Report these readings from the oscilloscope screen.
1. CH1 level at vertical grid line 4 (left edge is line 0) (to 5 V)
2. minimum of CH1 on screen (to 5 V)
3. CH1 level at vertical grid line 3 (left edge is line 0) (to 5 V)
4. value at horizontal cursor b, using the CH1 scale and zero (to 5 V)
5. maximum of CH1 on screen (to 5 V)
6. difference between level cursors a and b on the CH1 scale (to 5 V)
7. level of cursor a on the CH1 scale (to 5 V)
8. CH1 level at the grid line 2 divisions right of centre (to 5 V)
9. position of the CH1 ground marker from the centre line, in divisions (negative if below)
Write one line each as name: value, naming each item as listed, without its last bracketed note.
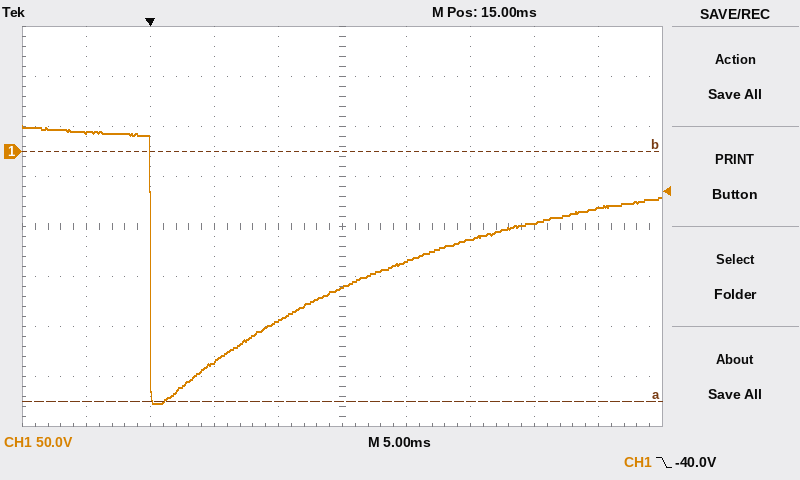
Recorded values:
CH1 level at vertical grid line 4 (left edge is line 0): -170 V
minimum of CH1 on screen: -250 V
CH1 level at vertical grid line 3 (left edge is line 0): -210 V
value at horizontal cursor b, using the CH1 scale and zero: 0 V
maximum of CH1 on screen: 25 V
difference between level cursors a and b on the CH1 scale: 250 V
level of cursor a on the CH1 scale: -250 V
CH1 level at the grid line 2 divisions right of centre: -90 V
position of the CH1 ground marker from the centre line, in divisions: +1.5 div
